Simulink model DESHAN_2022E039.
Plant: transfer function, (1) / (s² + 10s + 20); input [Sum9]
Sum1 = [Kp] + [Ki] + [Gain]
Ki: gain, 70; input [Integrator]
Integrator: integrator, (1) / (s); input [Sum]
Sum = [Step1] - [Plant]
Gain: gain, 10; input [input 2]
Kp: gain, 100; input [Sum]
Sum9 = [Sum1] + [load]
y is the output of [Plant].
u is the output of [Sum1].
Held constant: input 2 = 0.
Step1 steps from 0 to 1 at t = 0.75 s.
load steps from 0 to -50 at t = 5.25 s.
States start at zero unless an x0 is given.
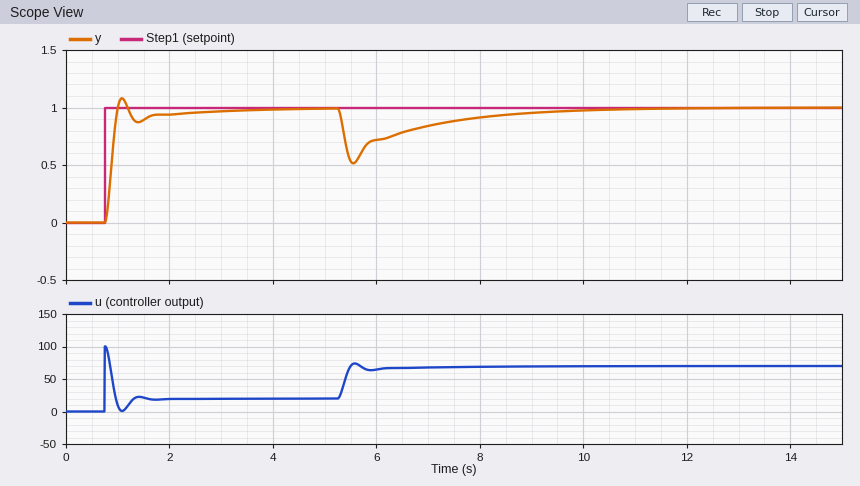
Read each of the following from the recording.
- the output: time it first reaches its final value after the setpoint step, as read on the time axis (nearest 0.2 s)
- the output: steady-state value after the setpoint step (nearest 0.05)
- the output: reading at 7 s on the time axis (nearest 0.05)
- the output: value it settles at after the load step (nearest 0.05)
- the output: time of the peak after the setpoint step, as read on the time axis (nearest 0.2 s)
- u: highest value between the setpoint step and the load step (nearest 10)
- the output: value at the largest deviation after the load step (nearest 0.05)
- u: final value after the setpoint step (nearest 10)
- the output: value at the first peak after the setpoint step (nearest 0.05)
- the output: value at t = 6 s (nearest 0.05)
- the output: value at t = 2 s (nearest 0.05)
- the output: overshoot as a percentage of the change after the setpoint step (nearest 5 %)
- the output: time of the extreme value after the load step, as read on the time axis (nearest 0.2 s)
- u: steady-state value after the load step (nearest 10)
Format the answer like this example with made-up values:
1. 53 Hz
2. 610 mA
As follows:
1. 1.0 s
2. 1.00
3. 0.85
4. 1.00
5. 1.0 s
6. 100
7. 0.50
8. 20
9. 1.10
10. 0.70
11. 0.95
12. 10 %
13. 5.6 s
14. 70
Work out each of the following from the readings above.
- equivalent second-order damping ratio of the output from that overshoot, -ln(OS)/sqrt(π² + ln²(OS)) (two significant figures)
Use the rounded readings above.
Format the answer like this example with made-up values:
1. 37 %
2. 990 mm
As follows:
1. 0.59
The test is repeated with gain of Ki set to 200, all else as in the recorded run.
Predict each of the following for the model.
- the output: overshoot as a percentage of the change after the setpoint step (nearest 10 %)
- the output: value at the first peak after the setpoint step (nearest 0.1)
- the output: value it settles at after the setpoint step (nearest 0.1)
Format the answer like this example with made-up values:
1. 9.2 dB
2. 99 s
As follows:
1. 20 %
2. 1.2
3. 1.0
